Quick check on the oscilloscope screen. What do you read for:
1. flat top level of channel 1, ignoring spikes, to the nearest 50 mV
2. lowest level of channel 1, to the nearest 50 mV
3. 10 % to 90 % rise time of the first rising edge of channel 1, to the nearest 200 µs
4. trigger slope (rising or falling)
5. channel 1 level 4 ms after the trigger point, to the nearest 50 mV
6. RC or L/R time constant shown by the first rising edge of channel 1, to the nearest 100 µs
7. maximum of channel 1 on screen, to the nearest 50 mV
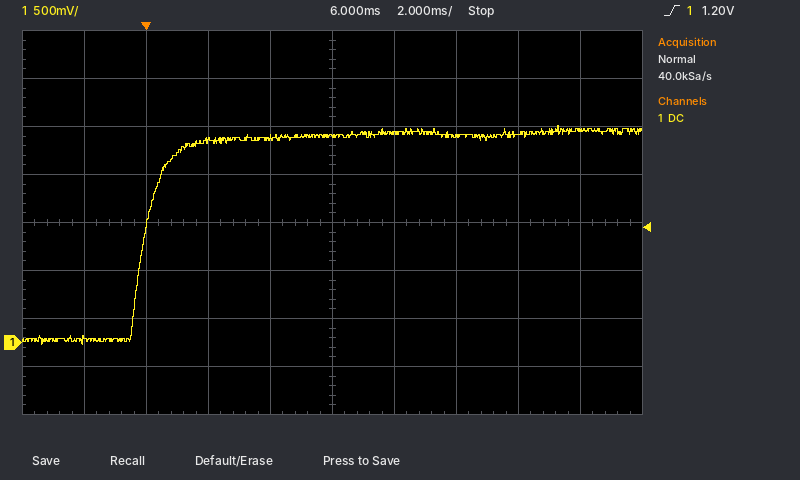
2.15 V
0 mV
1.4 ms
rising
2.15 V
600 µs
2.25 V
